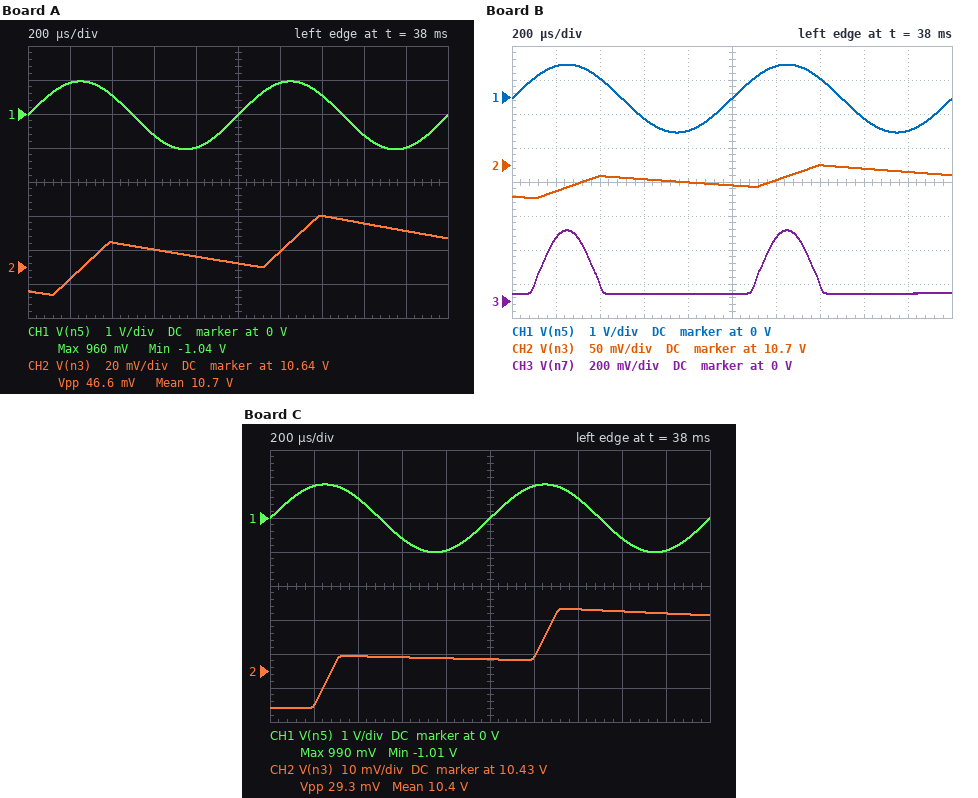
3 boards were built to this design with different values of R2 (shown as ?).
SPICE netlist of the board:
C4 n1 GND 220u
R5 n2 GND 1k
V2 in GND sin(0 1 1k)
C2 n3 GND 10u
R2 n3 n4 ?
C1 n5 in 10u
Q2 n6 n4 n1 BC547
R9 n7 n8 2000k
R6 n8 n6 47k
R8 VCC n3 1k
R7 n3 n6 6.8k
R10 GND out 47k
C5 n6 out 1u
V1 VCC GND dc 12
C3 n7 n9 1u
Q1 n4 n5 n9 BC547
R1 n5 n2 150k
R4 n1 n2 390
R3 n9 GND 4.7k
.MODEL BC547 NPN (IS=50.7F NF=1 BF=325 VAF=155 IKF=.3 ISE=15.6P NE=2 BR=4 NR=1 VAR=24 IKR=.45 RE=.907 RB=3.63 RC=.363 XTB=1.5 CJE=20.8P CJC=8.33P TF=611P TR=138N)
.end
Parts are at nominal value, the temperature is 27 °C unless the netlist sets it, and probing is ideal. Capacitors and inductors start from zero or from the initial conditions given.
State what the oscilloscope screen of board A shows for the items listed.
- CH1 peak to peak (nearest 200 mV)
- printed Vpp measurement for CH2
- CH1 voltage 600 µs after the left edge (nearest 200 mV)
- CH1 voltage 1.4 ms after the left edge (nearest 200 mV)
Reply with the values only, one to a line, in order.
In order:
2.0 V
46.6 mV
-600 mV
600 mV
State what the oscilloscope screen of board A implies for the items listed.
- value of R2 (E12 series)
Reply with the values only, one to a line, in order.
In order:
390 kΩ
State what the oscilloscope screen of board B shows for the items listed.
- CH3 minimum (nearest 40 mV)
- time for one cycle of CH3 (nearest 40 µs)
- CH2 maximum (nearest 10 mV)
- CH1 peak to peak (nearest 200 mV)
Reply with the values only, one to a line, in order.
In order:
40 mV
1.00 ms
10.70 V
2.0 V
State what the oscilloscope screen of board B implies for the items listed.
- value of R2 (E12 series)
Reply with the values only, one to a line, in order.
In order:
560 kΩ
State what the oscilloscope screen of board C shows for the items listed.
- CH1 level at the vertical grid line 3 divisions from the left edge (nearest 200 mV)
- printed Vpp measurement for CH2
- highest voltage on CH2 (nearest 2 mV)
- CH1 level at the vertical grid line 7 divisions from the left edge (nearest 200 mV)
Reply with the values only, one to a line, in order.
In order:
-600 mV
29.3 mV
10.448 V
600 mV
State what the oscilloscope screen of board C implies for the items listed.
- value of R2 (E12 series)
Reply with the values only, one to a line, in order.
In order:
120 kΩ
